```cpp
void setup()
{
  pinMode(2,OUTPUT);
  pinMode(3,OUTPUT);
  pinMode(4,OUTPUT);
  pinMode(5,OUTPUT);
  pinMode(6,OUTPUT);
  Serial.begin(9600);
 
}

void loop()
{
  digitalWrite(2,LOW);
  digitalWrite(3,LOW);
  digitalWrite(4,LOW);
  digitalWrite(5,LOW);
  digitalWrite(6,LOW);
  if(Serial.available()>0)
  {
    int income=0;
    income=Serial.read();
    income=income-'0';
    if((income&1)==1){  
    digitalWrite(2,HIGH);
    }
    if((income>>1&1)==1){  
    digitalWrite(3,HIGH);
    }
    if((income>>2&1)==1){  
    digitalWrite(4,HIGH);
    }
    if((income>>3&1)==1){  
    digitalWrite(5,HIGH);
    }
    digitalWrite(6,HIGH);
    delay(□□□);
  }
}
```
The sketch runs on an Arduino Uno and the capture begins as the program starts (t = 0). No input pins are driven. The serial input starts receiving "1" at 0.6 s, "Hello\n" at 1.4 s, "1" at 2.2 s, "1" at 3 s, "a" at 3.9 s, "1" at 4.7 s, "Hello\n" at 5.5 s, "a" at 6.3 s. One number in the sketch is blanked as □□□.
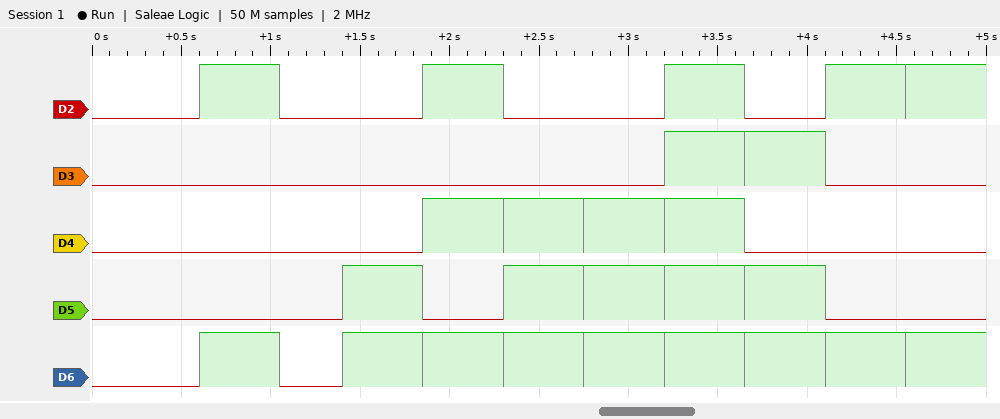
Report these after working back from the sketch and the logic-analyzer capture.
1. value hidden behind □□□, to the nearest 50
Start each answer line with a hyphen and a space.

- 450
